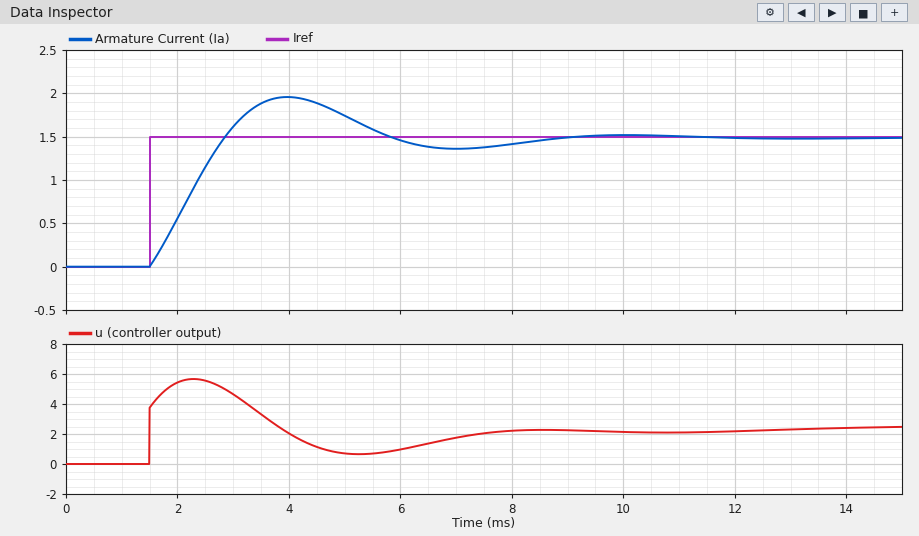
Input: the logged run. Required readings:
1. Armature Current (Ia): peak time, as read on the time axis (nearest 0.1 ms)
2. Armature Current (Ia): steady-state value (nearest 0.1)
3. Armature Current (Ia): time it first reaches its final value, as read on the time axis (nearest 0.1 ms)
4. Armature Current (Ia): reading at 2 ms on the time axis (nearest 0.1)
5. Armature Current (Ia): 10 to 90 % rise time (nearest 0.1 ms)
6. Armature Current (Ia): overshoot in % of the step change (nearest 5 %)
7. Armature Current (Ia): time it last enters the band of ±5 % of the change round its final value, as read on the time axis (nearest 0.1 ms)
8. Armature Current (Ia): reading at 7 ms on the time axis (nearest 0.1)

4.0 ms
1.5
2.8 ms
0.6
1.0 ms
30 %
8.0 ms
1.4
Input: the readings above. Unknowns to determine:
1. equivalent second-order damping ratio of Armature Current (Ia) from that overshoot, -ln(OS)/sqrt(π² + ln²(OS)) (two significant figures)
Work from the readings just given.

0.36
